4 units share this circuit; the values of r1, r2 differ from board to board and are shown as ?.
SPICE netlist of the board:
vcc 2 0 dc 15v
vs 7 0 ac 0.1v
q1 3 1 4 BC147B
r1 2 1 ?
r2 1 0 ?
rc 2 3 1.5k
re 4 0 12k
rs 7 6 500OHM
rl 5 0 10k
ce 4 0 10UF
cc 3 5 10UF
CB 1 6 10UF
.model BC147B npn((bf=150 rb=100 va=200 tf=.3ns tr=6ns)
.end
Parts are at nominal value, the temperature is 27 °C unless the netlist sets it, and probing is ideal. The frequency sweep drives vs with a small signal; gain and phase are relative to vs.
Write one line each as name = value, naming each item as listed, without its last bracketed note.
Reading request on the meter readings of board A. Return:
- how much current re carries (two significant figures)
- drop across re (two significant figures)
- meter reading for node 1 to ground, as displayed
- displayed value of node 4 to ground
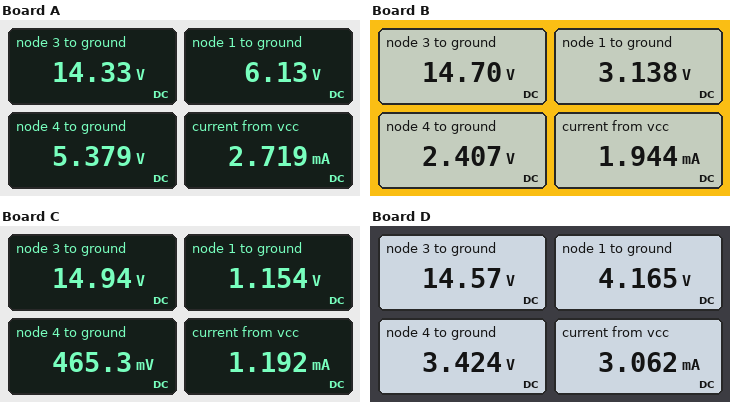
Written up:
how much current re carries = 450 µA
drop across re = 5.4 V
meter reading for node 1 to ground, as displayed = 6.13 V
displayed value of node 4 to ground = 5.379 V
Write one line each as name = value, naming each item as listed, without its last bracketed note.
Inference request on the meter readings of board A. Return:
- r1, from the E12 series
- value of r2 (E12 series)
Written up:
r1, from the E12 series = 3.9 kΩ
value of r2 = 2.7 kΩ
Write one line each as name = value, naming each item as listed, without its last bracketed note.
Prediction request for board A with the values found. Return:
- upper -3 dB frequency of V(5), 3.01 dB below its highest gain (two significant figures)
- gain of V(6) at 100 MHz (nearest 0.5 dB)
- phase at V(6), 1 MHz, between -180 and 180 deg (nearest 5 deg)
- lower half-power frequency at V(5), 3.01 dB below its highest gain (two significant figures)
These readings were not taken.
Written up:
upper -3 dB frequency of V(5), 3.01 dB below its highest gain = 68 MHz
gain of V(6) at 100 MHz = -7.5 dB
phase at V(6), 1 MHz, between -180 and 180 deg = 0 deg
lower half-power frequency at V(5), 3.01 dB below its highest gain = 260 Hz
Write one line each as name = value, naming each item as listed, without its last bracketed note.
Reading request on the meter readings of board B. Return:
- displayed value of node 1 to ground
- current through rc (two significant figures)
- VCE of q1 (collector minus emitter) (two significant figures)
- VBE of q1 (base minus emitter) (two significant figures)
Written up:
displayed value of node 1 to ground = 3.138 V
current through rc = 200 µA
VCE of q1 (collector minus emitter) = 12 V
VBE of q1 (base minus emitter) = 730 mV
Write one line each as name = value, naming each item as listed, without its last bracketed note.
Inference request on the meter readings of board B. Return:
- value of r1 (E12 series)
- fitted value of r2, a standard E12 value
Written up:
value of r1 = 6.8 kΩ
fitted value of r2, a standard E12 value = 1.8 kΩ
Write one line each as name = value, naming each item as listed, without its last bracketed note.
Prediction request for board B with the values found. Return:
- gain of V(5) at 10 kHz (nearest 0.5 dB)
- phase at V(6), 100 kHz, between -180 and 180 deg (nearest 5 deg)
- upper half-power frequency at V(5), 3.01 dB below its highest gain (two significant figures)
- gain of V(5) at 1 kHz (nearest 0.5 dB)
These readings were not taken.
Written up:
gain of V(5) at 10 kHz = 17.0 dB
phase at V(6), 100 kHz, between -180 and 180 deg = 0 deg
upper half-power frequency at V(5), 3.01 dB below its highest gain = 150 MHz
gain of V(5) at 1 kHz = 17.0 dB
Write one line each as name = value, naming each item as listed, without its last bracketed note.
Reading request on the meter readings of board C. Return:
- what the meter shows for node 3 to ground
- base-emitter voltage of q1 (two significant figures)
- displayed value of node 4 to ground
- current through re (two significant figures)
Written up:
what the meter shows for node 3 to ground = 14.94 V
base-emitter voltage of q1 = 690 mV
displayed value of node 4 to ground = 465.3 mV
current through re = 39 µA
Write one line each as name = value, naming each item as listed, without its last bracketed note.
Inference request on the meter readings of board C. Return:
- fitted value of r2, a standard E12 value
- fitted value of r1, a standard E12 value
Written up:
fitted value of r2, a standard E12 value = 1 kΩ
fitted value of r1, a standard E12 value = 12 kΩ
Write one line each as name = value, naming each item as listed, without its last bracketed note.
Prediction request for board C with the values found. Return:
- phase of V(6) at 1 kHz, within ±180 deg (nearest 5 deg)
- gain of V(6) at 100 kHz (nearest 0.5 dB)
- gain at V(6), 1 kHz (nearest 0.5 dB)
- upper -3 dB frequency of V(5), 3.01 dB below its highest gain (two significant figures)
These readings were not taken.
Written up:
phase of V(6) at 1 kHz, within ±180 deg = 0 deg
gain of V(6) at 100 kHz = -4.0 dB
gain at V(6), 1 kHz = -4.0 dB
upper -3 dB frequency of V(5), 3.01 dB below its highest gain = 840 MHz
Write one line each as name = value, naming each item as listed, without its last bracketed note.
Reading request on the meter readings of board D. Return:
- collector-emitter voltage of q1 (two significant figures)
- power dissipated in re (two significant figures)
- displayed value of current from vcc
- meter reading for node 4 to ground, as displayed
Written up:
collector-emitter voltage of q1 = 11 V
power dissipated in re = 980 µW
displayed value of current from vcc = 3.062 mA
meter reading for node 4 to ground, as displayed = 3.424 V
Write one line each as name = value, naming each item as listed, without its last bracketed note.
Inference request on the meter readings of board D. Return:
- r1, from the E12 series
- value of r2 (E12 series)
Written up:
r1, from the E12 series = 3.9 kΩ
value of r2 = 1.5 kΩ
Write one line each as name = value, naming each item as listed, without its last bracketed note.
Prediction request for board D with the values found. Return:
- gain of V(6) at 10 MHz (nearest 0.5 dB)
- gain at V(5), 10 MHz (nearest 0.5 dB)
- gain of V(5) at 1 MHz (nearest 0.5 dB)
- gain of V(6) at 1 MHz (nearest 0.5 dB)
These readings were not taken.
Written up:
gain of V(6) at 10 MHz = -3.5 dB
gain at V(5), 10 MHz = 19.5 dB
gain of V(5) at 1 MHz = 19.5 dB
gain of V(6) at 1 MHz = -3.5 dB
